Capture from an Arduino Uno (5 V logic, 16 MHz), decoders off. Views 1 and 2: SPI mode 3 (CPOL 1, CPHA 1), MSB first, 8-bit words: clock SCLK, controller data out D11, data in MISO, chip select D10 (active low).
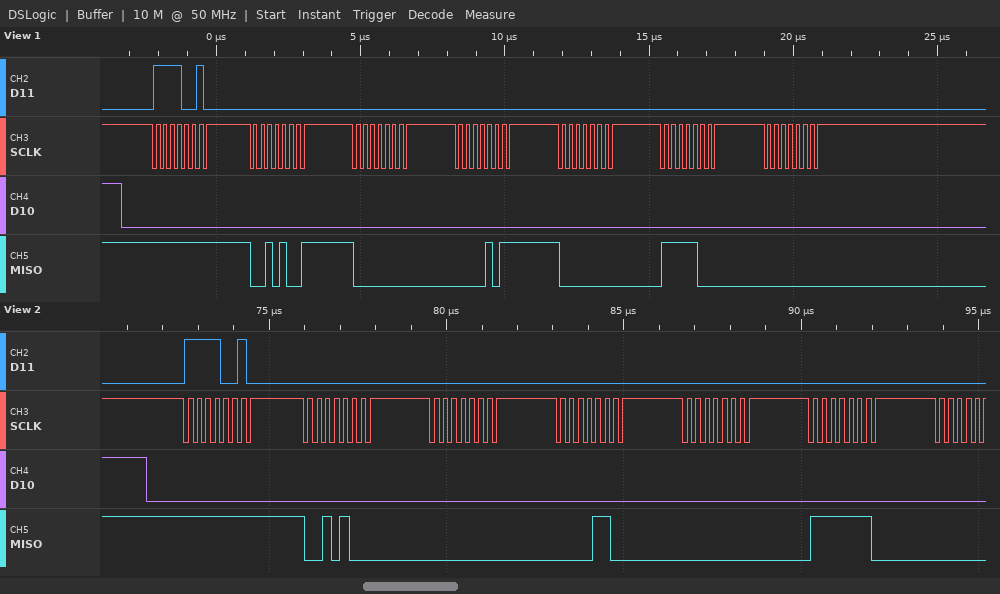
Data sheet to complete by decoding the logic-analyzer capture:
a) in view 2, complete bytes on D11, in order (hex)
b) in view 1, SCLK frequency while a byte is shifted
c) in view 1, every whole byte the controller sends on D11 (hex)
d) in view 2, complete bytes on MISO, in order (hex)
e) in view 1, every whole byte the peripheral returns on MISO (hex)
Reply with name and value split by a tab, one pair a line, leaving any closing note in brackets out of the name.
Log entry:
in view 2, complete bytes on D11, in order	F2 00 00 00 00 00
in view 1, SCLK frequency while a byte is shifted	4 MHz
in view 1, every whole byte the controller sends on D11	0xF2 0x00 0x00 0x00 0x00 0x00 0x00
in view 2, complete bytes on MISO, in order	FF 28 00 0C 00 FE
in view 1, every whole byte the peripheral returns on MISO	0xFF 0x29 0x00 0x0B 0x00 0xF8 0x00
